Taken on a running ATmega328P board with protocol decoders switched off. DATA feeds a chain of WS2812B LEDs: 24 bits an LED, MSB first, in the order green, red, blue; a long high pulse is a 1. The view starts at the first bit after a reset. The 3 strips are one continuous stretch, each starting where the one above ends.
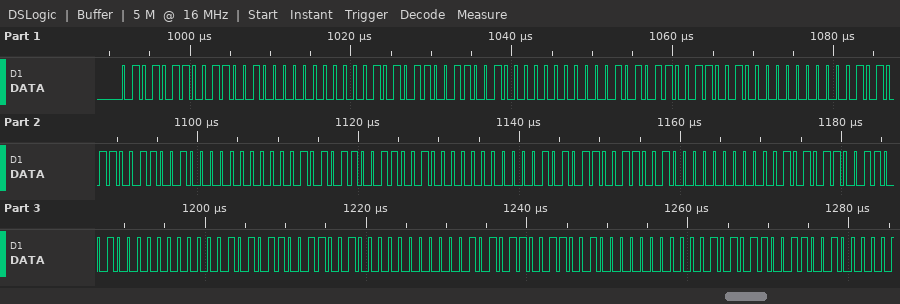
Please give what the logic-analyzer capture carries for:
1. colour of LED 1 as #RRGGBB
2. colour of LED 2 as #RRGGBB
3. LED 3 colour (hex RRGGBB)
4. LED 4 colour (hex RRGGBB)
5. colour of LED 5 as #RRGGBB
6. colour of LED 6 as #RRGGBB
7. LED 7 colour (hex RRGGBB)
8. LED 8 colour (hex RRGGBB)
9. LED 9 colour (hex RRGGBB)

#645600
#645600
#645600
#645600
#645600
#645600
#645600
#645600
#645600
